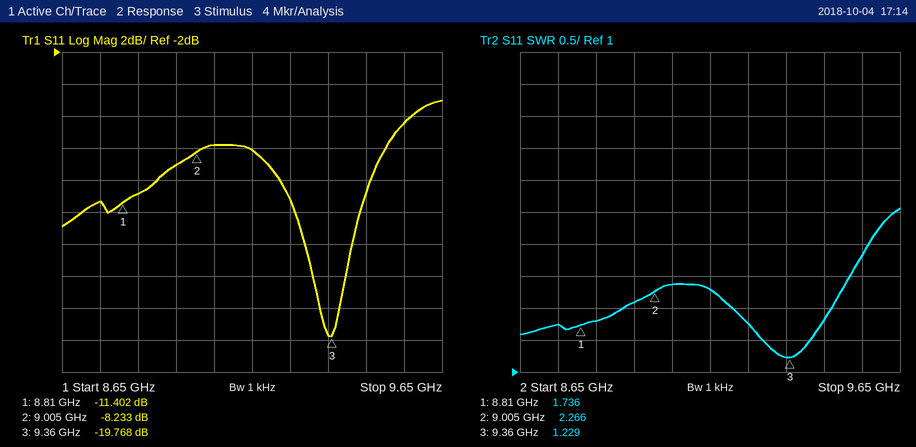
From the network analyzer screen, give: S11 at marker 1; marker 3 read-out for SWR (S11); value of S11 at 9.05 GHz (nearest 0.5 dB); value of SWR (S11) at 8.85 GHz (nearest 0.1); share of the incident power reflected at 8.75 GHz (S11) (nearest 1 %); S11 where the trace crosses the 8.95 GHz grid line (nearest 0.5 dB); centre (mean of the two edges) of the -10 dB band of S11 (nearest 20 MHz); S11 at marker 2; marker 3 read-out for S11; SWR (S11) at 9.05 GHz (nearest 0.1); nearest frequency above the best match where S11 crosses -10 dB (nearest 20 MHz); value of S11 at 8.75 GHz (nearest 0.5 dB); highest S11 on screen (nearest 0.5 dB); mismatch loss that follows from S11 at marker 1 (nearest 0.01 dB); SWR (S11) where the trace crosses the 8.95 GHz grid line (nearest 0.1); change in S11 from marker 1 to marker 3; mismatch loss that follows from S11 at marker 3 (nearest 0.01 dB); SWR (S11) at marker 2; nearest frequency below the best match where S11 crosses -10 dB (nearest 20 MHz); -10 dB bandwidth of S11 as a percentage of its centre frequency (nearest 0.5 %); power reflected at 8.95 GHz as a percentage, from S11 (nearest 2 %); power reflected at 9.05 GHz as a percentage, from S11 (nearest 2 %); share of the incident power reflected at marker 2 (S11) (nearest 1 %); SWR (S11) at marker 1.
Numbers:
-11.402 dB
1.229
-8.0 dB
1.8
7 %
-9.0 dB
9.34 GHz
-8.233 dB
-19.768 dB
2.4
9.46 GHz
-11.5 dB
-5.0 dB
0.33 dB
2.1
-8.366 dB
0.05 dB
2.266
9.22 GHz
2.5 %
12 %
16 %
15 %
1.736
